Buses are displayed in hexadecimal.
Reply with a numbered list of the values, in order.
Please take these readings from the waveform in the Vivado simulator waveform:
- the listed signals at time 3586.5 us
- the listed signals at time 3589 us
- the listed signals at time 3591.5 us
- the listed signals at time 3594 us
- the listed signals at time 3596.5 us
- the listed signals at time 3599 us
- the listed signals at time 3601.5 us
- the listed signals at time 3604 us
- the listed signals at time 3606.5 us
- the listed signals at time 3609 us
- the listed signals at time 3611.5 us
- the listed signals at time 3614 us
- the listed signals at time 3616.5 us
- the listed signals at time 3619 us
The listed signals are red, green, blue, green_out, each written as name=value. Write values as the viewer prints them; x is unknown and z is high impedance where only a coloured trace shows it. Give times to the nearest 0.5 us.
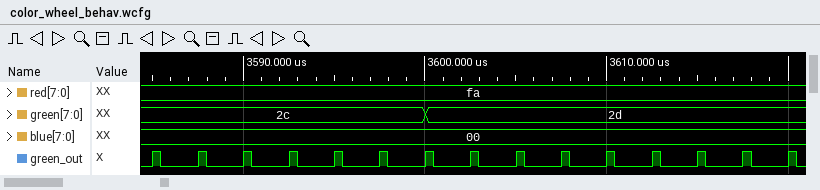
1. red=fa, green=2c, blue=00, green_out=0
2. red=fa, green=2c, blue=00, green_out=0
3. red=fa, green=2c, blue=00, green_out=0
4. red=fa, green=2c, blue=00, green_out=0
5. red=fa, green=2c, blue=00, green_out=0
6. red=fa, green=2c, blue=00, green_out=0
7. red=fa, green=2d, blue=00, green_out=0
8. red=fa, green=2d, blue=00, green_out=0
9. red=fa, green=2d, blue=00, green_out=0
10. red=fa, green=2d, blue=00, green_out=0
11. red=fa, green=2d, blue=00, green_out=0
12. red=fa, green=2d, blue=00, green_out=0
13. red=fa, green=2d, blue=00, green_out=0
14. red=fa, green=2d, blue=00, green_out=0
